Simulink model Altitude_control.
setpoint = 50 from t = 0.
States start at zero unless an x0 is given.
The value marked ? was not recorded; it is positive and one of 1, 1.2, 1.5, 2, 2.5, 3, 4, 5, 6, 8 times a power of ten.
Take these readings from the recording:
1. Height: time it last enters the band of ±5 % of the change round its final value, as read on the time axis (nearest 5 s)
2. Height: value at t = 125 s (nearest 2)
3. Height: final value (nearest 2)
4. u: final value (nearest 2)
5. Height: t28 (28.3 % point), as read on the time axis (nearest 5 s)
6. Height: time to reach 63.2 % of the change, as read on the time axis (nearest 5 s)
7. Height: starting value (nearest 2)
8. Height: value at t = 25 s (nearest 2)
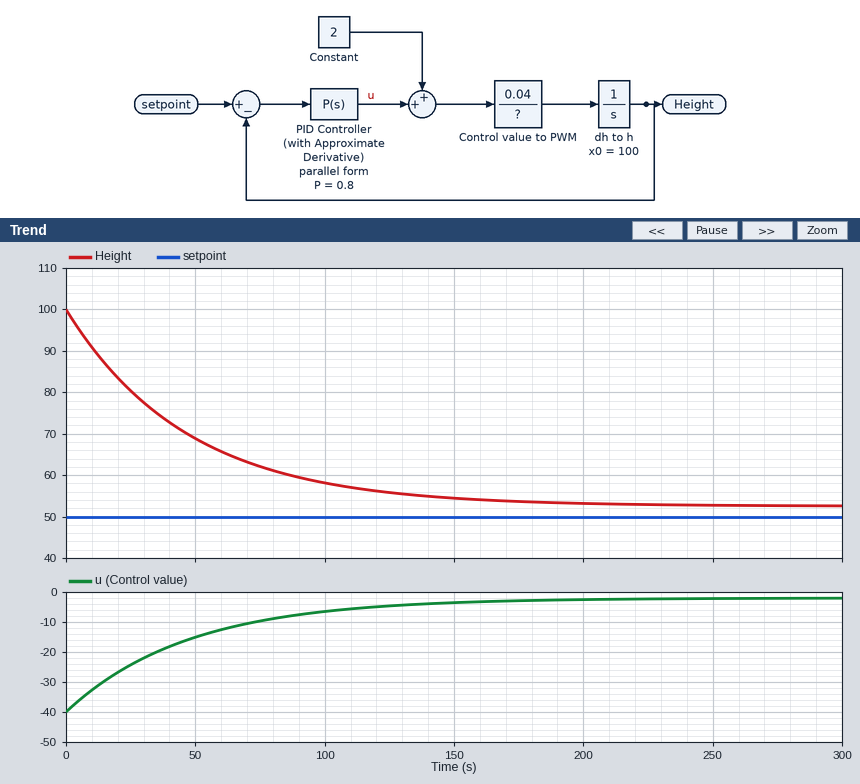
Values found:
140 s
56
52
-2
15 s
45 s
100
80
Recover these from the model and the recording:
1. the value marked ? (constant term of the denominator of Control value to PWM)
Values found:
1.5
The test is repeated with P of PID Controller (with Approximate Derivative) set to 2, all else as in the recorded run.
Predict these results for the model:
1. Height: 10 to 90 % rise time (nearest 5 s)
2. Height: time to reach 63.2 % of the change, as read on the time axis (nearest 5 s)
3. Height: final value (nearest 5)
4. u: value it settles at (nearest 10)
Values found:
40 s
20 s
50
0
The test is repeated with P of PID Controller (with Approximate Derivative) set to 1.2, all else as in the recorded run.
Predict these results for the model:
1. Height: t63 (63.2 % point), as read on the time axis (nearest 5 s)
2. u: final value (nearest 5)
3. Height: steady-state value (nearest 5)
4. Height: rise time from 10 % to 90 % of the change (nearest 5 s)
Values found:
30 s
0
50
70 s
